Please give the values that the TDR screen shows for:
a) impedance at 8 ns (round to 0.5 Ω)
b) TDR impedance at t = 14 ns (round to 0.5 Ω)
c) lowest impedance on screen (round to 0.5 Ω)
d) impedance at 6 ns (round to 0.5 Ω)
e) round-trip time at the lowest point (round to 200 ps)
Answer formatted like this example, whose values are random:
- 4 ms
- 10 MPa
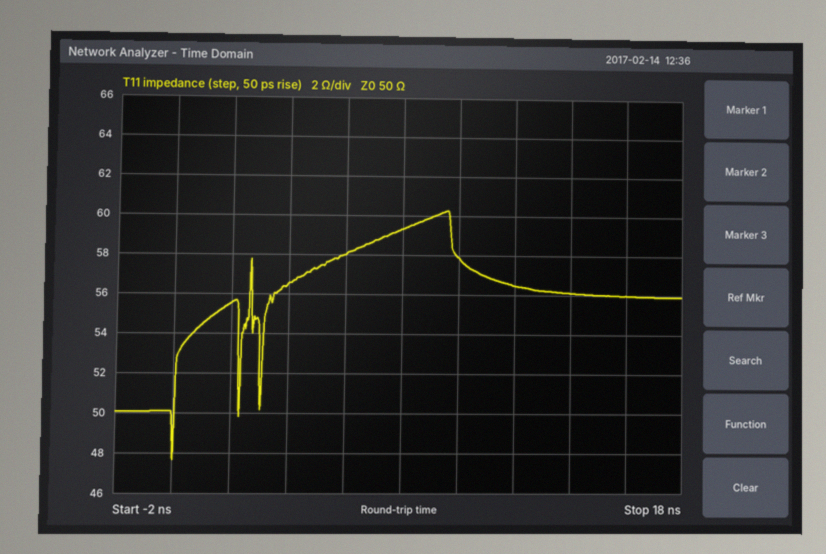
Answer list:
- 59.5 Ω
- 56.0 Ω
- 47.5 Ω
- 58.0 Ω
- 0.0 ns
